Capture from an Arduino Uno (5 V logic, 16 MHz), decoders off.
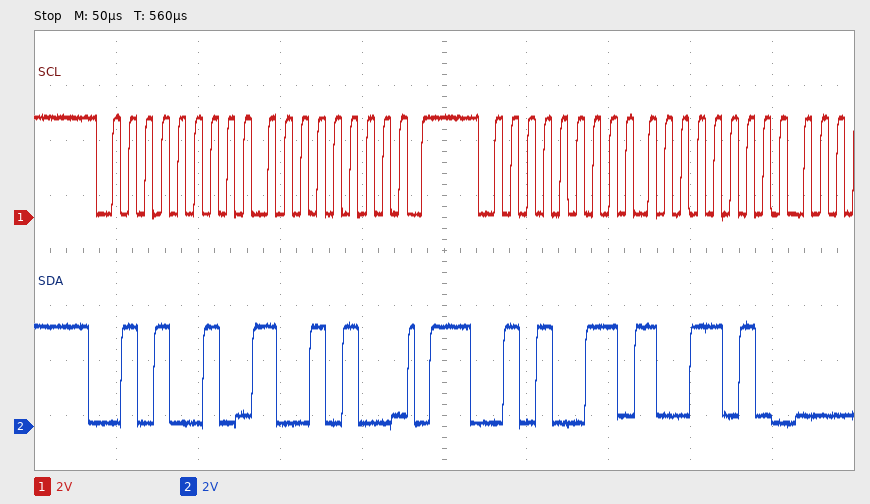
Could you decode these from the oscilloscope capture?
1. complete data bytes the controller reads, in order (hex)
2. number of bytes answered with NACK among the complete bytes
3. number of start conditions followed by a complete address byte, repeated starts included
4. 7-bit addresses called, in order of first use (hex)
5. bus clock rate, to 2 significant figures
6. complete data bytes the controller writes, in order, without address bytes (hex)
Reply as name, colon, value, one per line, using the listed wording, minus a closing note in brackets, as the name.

complete data bytes the controller reads, in order: 9A
number of bytes answered with NACK among the complete bytes: 0
number of start conditions followed by a complete address byte, repeated starts included: 2
7-bit addresses called, in order of first use: 0x29
bus clock rate, to 2 significant figures: 100 kHz
complete data bytes the controller writes, in order, without address bytes: 94
